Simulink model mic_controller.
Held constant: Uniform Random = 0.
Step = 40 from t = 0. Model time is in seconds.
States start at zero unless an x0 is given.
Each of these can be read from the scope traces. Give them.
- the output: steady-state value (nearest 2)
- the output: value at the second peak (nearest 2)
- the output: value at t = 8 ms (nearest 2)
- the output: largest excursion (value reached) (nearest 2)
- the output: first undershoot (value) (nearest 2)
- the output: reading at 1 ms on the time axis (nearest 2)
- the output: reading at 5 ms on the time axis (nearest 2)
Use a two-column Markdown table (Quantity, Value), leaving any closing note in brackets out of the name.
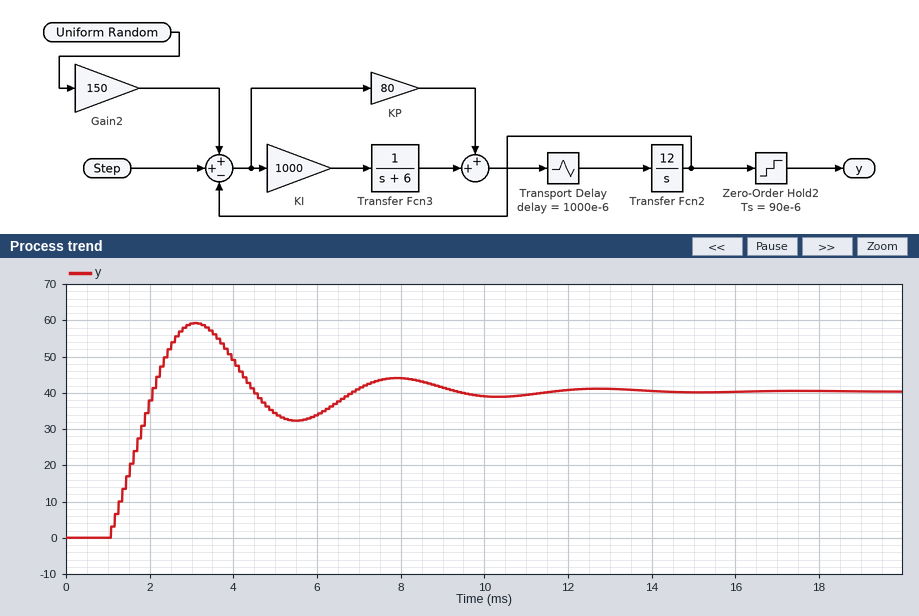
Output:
| Quantity | Value |
|---|---|
| the output: steady-state value | 40 |
| the output: value at the second peak | 44 |
| the output: value at t = 8 ms | 44 |
| the output: largest excursion (value reached) | 60 |
| the output: first undershoot (value) | 32 |
| the output: reading at 1 ms on the time axis | 0 |
| the output: reading at 5 ms on the time axis | 34 |
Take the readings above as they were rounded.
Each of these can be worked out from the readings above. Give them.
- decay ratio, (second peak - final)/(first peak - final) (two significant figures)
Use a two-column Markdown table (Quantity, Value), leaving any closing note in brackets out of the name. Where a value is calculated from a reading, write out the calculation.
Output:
| Quantity | Value |
|---|---|
| decay ratio, (second peak - final)/(first peak - final) | (44 - 40) / (60 - 40) = 0.20 |
